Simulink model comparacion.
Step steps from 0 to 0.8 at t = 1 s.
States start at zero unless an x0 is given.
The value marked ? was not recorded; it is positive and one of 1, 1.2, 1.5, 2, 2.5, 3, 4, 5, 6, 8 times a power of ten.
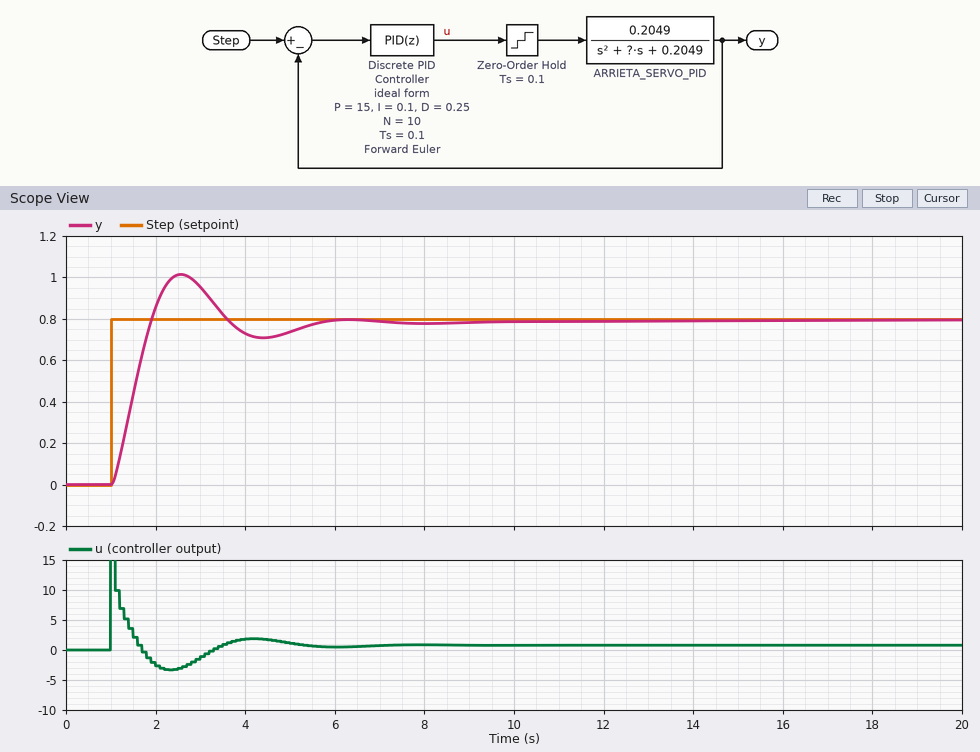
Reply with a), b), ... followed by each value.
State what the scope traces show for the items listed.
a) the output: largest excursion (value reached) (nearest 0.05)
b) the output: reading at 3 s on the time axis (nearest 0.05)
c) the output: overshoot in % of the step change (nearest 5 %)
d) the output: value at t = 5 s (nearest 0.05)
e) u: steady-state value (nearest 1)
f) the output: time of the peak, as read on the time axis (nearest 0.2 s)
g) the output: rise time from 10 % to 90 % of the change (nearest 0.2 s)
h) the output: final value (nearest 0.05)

a) 1.00
b) 0.95
c) 25 %
d) 0.75
e) 1
f) 2.6 s
g) 0.6 s
h) 0.80
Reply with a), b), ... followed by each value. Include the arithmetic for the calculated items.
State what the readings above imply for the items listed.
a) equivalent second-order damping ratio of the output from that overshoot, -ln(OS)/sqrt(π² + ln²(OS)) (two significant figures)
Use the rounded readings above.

a) ln(0.25) = -1.386; 1.386 / sqrt(9.870 + 1.922) = 0.40
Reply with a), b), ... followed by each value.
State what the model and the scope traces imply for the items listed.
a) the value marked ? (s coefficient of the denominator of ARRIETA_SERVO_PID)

a) 0.8
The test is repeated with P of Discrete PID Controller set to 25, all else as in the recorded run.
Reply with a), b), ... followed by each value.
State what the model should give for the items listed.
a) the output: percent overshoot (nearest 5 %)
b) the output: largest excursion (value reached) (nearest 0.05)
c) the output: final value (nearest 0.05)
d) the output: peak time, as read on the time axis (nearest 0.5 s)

a) 30 %
b) 1.05
c) 0.80
d) 2.0 s
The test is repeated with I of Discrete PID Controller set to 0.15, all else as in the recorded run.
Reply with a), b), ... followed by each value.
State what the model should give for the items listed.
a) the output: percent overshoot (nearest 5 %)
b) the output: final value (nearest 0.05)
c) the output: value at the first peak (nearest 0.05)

a) 30 %
b) 0.80
c) 1.05
